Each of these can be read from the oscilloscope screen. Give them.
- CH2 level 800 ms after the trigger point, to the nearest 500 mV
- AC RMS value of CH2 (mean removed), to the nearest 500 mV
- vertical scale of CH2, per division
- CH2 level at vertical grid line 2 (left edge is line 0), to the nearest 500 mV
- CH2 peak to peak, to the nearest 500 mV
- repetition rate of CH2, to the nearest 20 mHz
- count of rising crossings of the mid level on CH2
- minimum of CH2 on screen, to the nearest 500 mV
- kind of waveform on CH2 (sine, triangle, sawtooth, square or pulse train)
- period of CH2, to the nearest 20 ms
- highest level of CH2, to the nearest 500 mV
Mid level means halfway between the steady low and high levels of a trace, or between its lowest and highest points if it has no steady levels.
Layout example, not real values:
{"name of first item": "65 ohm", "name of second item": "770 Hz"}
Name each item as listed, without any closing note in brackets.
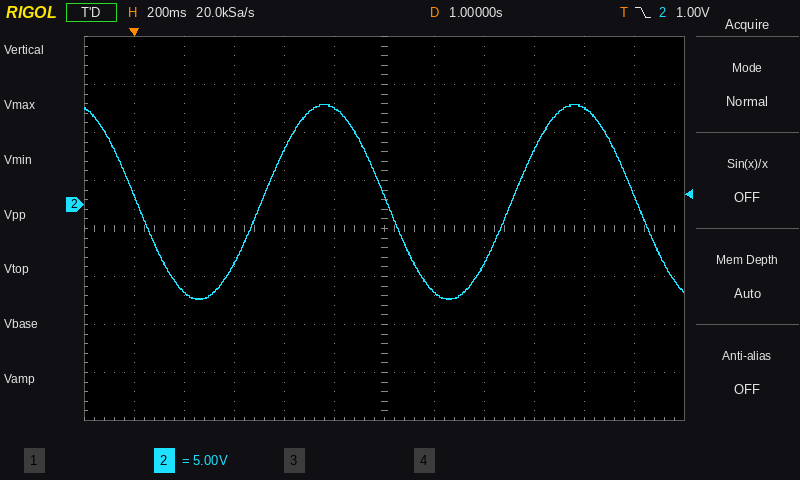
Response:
{"CH2 level 800 ms after the trigger point, to the nearest 500 mV": "10.0 V", "AC RMS value of CH2 (mean removed), to the nearest 500 mV": "7.0 V", "vertical scale of CH2, per division": "5 V", "CH2 level at vertical grid line 2 (left edge is line 0), to the nearest 500 mV": "-9.0 V", "CH2 peak to peak, to the nearest 500 mV": "20.5 V", "repetition rate of CH2, to the nearest 20 mHz": "1.00 Hz", "count of rising crossings of the mid level on CH2": "2", "minimum of CH2 on screen, to the nearest 500 mV": "-10.0 V", "kind of waveform on CH2": "sine", "period of CH2, to the nearest 20 ms": "1.00 s", "highest level of CH2, to the nearest 500 mV": "10.5 V"}
